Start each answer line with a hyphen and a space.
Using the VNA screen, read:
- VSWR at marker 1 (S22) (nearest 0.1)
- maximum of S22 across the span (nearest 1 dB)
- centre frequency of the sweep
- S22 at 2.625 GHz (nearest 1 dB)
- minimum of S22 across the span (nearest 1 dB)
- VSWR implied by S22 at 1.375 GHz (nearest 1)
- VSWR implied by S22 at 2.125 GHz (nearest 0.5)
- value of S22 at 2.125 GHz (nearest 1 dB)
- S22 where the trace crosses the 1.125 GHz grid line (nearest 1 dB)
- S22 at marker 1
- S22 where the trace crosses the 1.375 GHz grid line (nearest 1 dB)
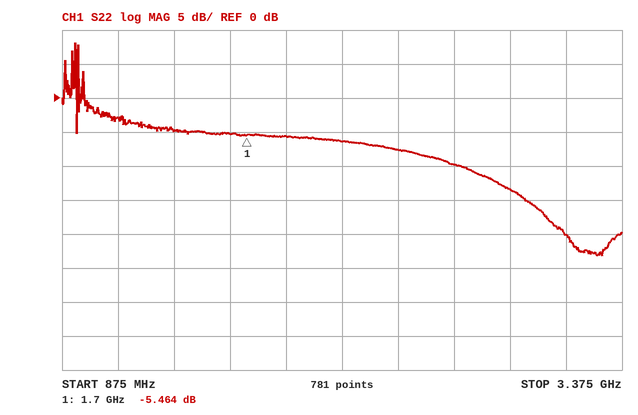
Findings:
- 3.3
- 8 dB
- 2.125 GHz
- -10 dB
- -23 dB
- 4
- 3.0
- -6 dB
- -3 dB
- -5.464 dB
- -5 dB
